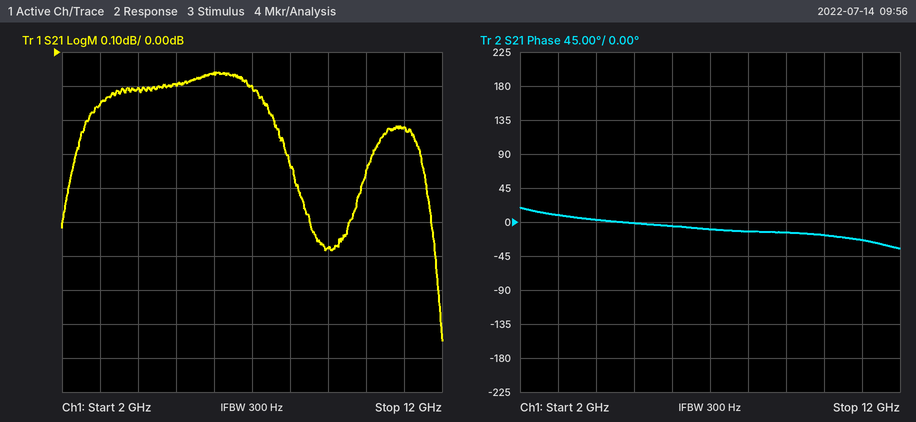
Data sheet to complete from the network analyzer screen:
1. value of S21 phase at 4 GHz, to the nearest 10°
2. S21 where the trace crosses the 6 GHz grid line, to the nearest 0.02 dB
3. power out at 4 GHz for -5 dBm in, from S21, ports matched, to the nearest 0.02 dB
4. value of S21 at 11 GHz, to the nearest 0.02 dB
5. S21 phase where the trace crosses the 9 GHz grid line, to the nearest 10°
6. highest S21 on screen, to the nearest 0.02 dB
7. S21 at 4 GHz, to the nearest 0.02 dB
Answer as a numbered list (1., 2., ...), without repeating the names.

1. 0°
2. -0.06 dB
3. -5.10 dBm
4. -0.22 dB
5. -10°
6. -0.06 dB
7. -0.10 dB
